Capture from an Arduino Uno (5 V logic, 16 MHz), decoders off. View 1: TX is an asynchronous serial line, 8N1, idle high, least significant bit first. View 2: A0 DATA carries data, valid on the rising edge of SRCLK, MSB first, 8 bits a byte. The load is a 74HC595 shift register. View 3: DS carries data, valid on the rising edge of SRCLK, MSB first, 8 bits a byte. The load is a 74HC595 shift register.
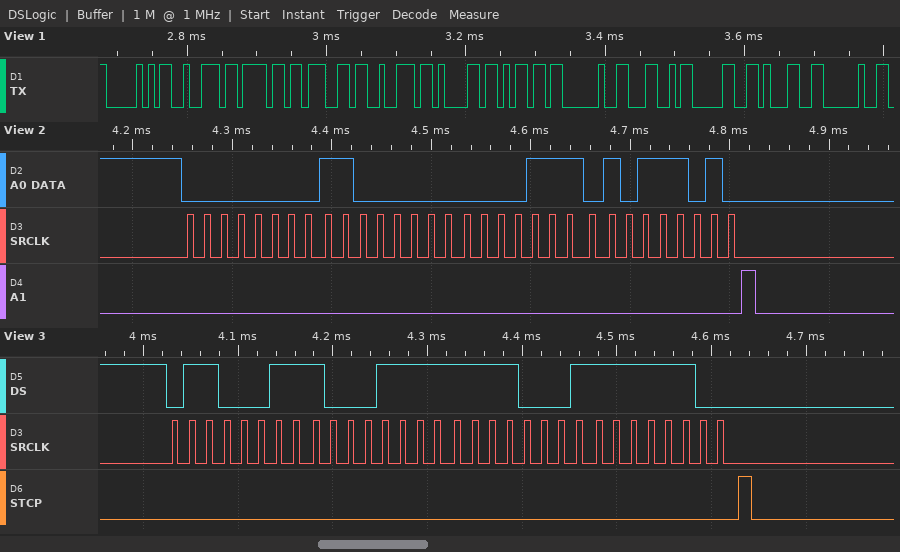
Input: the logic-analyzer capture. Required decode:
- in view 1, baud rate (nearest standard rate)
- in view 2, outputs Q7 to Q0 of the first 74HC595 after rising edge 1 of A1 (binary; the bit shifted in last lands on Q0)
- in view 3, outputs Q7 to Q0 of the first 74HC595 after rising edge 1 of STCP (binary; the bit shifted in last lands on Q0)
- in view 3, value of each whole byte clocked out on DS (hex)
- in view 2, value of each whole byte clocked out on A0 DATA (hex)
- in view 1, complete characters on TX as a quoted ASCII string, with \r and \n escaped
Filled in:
115200 baud
10111010
11111100
63 8F F1 FC
00 C0 0E BA
"Program L01 "
